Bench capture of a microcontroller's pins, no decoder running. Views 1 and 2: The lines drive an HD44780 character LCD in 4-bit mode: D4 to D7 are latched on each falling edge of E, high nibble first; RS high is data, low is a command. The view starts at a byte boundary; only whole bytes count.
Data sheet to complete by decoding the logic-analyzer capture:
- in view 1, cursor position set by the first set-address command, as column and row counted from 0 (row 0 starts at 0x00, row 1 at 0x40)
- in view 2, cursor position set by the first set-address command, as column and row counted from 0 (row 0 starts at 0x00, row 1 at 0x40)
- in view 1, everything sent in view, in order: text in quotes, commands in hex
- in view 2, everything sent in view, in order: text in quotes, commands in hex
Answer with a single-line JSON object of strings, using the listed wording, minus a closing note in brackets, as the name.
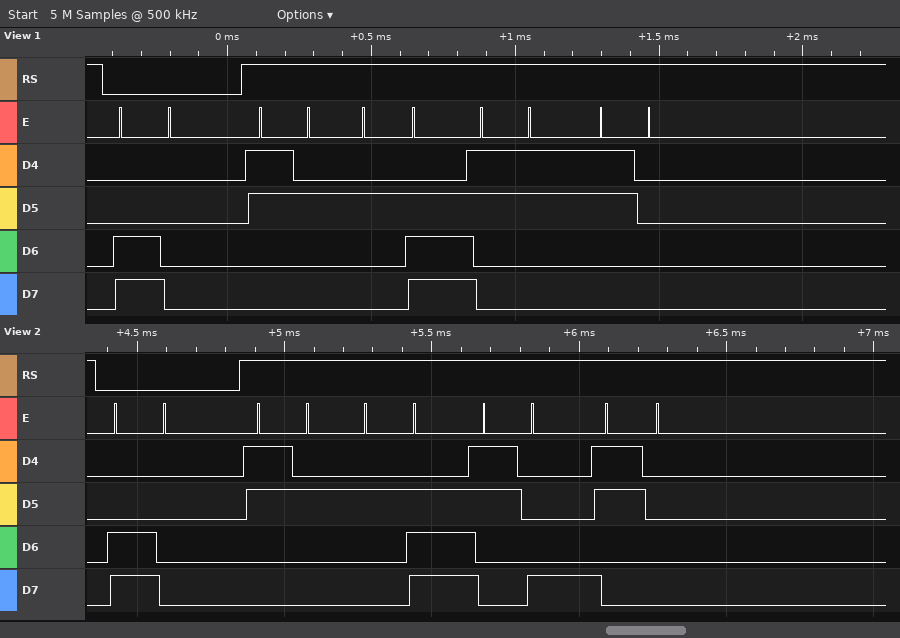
{"in view 1, cursor position set by the first set-address command, as column and row counted from 0": "column 0, row 1", "in view 2, cursor position set by the first set-address command, as column and row counted from 0": "column 0, row 1", "in view 1, everything sent in view, in order: text in quotes, commands in hex": "0xC0 \"2.30\"", "in view 2, everything sent in view, in order: text in quotes, commands in hex": "0xC0 \"2.80\""}
